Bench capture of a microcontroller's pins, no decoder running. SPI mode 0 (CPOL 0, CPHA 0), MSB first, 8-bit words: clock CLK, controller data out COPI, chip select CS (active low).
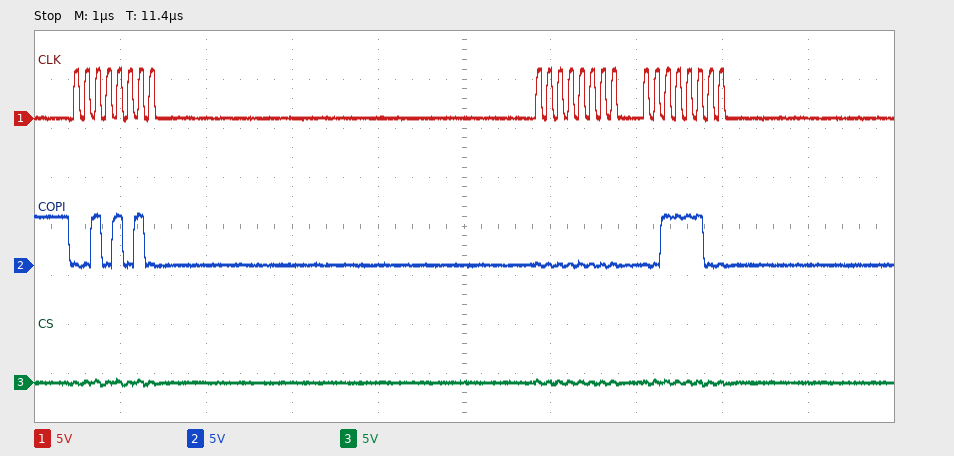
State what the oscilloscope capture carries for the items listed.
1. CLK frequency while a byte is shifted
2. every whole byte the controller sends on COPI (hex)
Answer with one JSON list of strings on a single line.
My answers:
["8 MHz", "2A 00 3C"]
